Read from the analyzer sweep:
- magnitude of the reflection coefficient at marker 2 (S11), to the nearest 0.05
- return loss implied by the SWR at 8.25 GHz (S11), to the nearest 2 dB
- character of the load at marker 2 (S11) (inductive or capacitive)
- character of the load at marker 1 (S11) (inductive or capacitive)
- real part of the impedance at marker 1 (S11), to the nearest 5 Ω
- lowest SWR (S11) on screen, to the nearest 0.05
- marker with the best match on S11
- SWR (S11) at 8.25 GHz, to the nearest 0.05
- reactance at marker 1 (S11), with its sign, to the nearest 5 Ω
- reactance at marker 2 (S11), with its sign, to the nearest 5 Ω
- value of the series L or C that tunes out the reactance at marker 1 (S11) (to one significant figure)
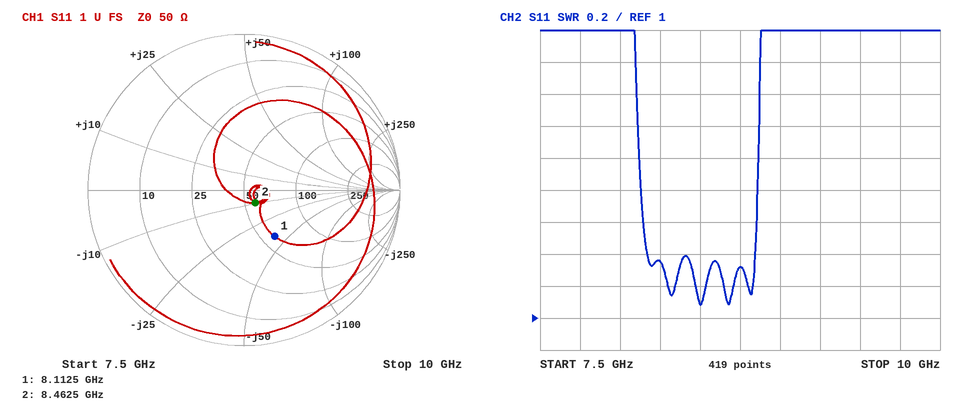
0.10
16 dB
capacitive
capacitive
60 Ω
1.10
marker 2
1.35
-40 Ω
-10 Ω
800 pH
